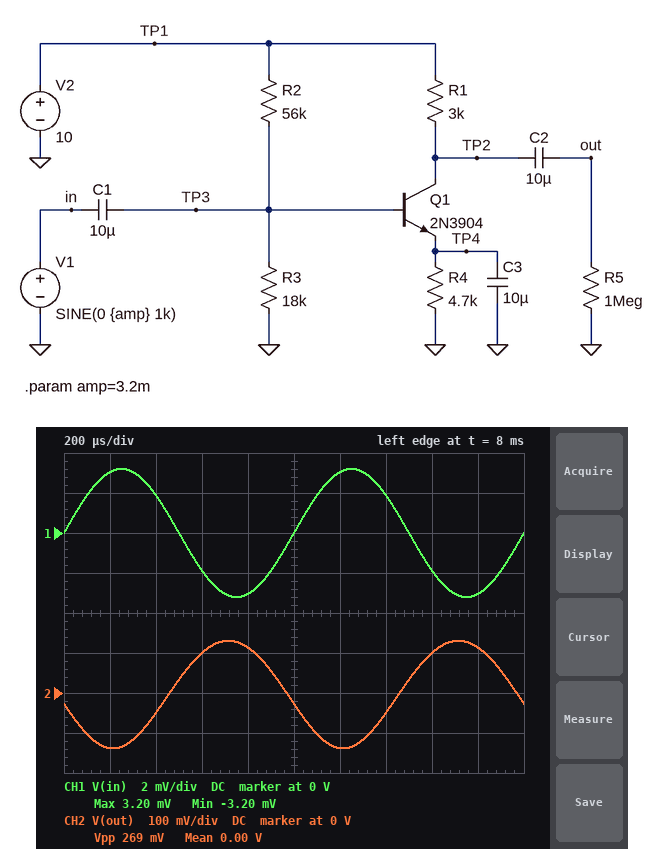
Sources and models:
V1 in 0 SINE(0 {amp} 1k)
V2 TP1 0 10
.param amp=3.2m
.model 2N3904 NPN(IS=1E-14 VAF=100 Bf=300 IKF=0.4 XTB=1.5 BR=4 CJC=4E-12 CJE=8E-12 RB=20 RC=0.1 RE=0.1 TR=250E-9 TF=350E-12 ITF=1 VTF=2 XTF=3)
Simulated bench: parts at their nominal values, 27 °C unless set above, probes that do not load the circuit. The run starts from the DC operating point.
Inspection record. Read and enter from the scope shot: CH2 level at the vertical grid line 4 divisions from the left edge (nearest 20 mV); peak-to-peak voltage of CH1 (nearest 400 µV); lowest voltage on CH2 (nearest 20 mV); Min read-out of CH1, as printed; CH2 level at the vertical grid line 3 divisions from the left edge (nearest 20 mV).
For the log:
120 mV
6.4 mV
-140 mV
-3.20 mV
100 mV
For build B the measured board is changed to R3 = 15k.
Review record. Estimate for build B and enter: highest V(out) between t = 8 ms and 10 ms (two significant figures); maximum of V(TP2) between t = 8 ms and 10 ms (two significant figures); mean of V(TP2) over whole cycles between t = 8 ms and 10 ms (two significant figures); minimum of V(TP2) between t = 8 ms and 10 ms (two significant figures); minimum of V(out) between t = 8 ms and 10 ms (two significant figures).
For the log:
110 mV
9.2 V
9.1 V
8.9 V
-120 mV
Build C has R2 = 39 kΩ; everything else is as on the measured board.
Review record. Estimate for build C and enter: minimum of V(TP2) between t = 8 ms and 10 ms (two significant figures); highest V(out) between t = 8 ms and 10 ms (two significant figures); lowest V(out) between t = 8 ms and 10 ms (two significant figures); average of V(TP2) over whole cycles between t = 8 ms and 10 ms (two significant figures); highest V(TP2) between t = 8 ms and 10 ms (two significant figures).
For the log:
8.2 V
180 mV
-190 mV
8.4 V
8.6 V
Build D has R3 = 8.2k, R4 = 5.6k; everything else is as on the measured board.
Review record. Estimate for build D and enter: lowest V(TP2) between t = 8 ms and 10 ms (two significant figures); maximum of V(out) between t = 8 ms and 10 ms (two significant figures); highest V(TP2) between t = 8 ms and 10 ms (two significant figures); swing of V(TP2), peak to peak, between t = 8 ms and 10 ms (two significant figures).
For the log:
9.6 V
43 mV
9.7 V
88 mV
